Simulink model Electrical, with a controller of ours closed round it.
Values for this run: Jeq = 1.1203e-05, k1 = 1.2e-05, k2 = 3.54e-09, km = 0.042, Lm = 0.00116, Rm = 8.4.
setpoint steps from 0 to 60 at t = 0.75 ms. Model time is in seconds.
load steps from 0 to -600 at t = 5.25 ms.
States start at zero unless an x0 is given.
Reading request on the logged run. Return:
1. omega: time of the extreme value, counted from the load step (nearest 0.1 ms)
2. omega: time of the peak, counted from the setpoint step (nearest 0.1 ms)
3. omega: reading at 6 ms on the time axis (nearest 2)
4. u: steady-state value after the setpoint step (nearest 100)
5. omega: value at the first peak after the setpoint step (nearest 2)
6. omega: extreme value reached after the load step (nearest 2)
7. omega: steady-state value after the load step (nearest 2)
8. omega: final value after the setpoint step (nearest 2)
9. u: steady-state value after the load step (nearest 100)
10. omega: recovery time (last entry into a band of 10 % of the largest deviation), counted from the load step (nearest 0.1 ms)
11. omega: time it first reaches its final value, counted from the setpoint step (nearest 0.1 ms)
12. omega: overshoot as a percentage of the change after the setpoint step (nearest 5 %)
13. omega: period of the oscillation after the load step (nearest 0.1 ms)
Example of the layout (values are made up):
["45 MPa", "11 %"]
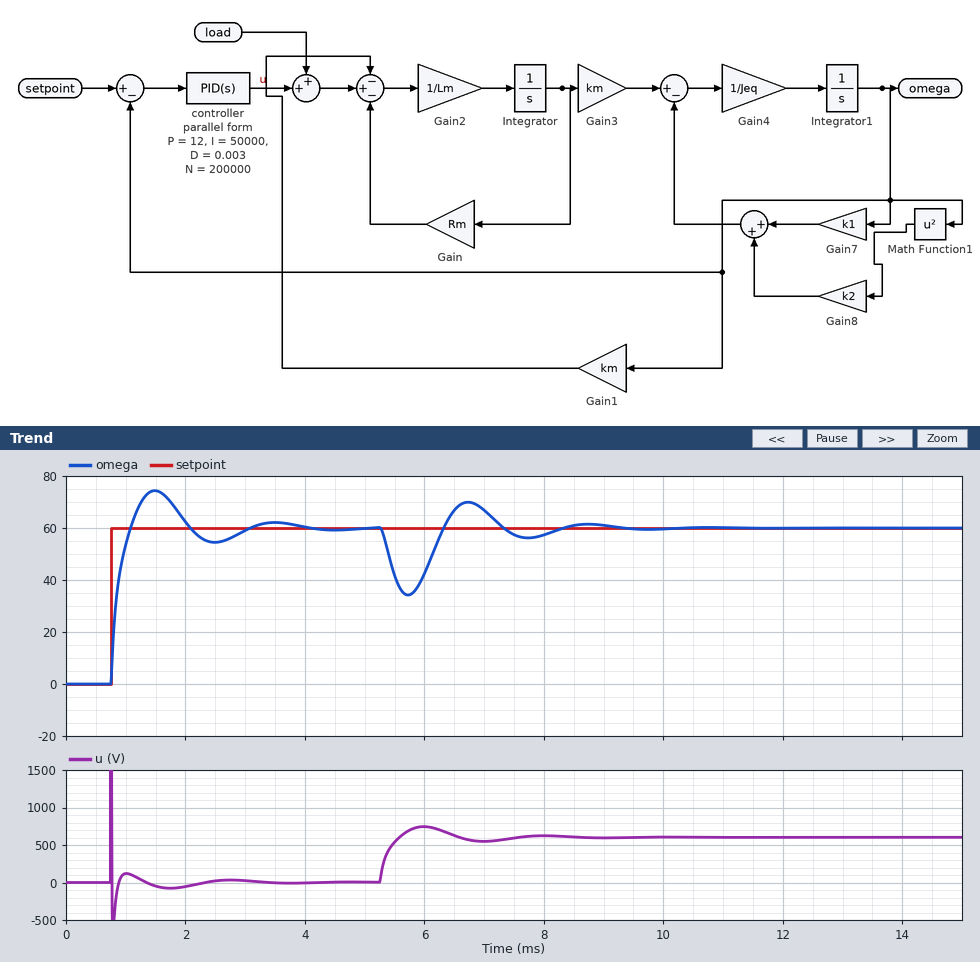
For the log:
["0.5 ms", "0.7 ms", "42", "0", "74", "34", "60", "60", "600", "2.8 ms", "0.3 ms", "25 %", "2.0 ms"]
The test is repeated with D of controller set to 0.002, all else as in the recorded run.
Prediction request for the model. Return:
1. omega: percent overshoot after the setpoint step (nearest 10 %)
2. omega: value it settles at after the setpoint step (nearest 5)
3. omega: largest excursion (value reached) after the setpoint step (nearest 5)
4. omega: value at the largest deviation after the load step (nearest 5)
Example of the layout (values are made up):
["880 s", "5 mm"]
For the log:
["30 %", "60", "80", "30"]
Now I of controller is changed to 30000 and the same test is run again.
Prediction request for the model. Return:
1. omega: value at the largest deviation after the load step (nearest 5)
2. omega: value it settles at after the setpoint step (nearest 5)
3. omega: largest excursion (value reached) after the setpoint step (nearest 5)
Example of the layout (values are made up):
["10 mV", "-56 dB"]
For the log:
["30", "60", "70"]
